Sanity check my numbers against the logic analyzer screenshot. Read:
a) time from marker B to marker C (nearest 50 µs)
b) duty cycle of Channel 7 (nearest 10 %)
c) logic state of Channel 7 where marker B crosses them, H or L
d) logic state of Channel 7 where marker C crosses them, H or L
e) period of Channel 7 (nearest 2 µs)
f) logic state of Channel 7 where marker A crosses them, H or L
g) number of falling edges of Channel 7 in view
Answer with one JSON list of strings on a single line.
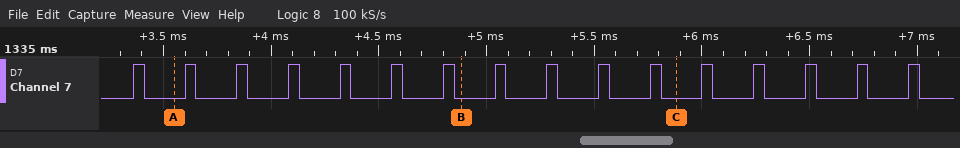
["1000 µs", "20 %", "Channel 7=L", "Channel 7=L", "240 µs", "Channel 7=L", "16"]
